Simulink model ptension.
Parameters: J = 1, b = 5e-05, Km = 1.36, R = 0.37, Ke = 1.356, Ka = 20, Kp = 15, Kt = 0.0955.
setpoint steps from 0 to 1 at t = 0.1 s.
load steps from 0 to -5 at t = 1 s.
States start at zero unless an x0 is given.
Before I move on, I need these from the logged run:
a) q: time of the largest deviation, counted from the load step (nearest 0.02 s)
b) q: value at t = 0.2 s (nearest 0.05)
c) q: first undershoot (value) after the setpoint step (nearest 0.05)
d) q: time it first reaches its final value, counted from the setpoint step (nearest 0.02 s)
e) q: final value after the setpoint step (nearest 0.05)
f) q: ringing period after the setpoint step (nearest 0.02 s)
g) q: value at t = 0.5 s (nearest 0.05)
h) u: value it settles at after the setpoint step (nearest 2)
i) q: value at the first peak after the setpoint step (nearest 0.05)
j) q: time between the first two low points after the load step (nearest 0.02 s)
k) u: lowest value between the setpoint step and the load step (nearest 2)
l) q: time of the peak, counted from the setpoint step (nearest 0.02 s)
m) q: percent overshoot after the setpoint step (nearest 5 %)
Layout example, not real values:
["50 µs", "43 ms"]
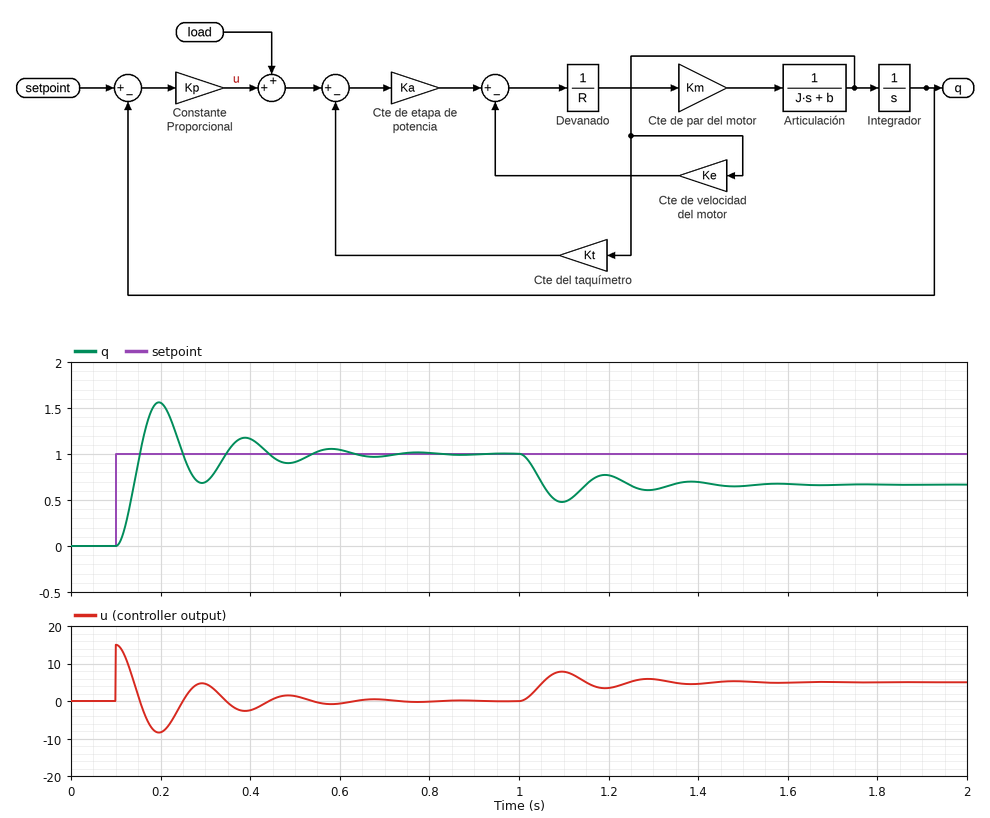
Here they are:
["0.10 s", "1.55", "0.70", "0.06 s", "1.00", "0.20 s", "0.90", "0", "1.55", "0.20 s", "-8", "0.10 s", "55 %"]
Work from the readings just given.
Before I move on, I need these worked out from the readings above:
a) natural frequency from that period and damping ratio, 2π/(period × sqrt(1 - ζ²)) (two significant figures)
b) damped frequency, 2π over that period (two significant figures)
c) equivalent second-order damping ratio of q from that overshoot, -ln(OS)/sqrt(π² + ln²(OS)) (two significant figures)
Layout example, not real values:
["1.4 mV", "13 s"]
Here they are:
["32 rad/s", "31 rad/s", "0.19"]
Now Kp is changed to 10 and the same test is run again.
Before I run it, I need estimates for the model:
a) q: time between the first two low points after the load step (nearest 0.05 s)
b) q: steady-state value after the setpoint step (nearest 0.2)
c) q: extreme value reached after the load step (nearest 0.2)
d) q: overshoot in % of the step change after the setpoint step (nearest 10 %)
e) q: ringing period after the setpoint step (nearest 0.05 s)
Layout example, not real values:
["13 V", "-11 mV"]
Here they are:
["0.25 s", "1.0", "0.2", "50 %", "0.25 s"]
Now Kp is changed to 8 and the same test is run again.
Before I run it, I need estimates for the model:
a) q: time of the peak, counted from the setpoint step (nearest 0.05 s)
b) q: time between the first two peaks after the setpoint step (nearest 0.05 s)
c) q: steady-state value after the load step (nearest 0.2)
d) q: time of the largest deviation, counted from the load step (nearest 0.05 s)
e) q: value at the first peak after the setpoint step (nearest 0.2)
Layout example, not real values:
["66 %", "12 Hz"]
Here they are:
["0.15 s", "0.25 s", "0.4", "0.15 s", "1.4"]
